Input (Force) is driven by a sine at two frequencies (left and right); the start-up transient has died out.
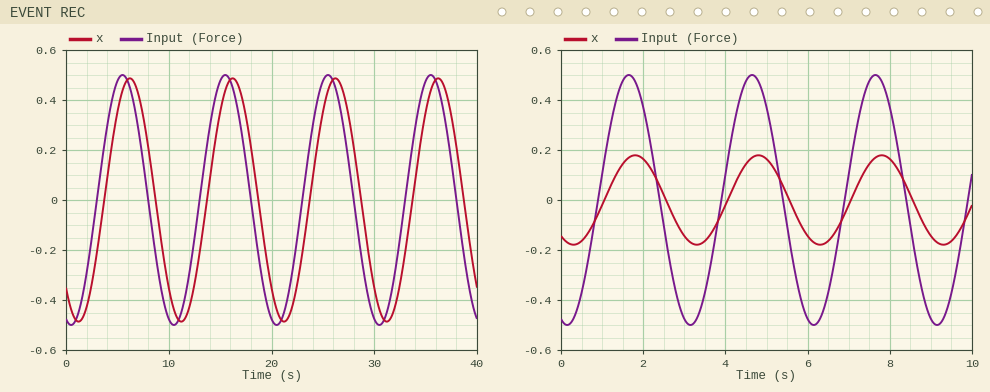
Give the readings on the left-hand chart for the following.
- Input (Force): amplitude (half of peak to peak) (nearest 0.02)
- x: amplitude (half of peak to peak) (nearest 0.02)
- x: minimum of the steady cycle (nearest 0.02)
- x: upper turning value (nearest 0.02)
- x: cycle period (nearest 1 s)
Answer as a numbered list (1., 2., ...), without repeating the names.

1. 0.50
2. 0.48
3. -0.48
4. 0.48
5. 10 s
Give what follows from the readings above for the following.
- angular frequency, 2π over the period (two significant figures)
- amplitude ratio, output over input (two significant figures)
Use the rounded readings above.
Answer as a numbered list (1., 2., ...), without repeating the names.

1. 0.63 rad/s
2. 0.96
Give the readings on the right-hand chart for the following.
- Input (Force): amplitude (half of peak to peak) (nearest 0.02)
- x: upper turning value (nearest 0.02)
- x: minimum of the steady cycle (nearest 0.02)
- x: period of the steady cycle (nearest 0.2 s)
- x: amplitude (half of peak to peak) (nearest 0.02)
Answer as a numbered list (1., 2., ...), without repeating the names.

1. 0.50
2. 0.18
3. -0.18
4. 3.0 s
5. 0.18
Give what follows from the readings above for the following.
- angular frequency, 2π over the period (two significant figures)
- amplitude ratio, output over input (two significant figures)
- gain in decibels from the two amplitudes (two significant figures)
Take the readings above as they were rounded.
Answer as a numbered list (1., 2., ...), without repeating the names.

1. 2.1 rad/s
2. 0.36
3. -8.9 dB
